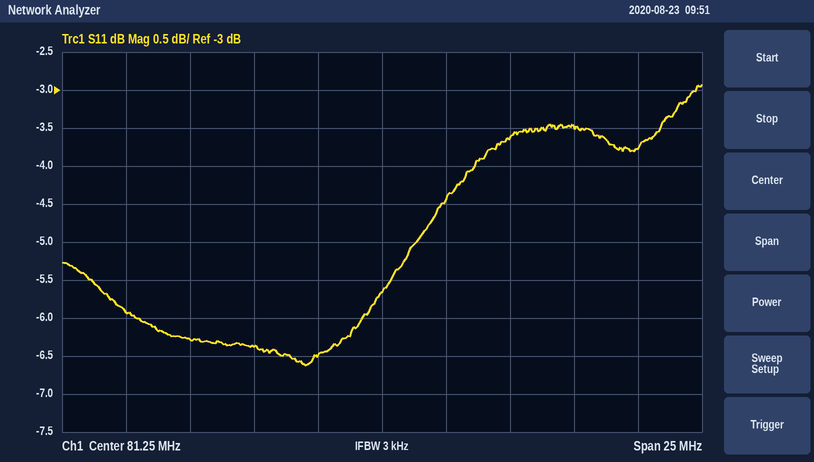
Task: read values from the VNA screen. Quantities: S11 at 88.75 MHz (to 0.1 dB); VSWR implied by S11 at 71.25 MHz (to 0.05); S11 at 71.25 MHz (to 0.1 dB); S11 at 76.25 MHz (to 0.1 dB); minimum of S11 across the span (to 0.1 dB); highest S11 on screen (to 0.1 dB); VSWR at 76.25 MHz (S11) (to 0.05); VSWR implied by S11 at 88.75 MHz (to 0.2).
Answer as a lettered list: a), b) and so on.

a) -3.5 dB
b) 3.05
c) -5.9 dB
d) -6.4 dB
e) -6.6 dB
f) -2.9 dB
g) 2.85
h) 5.0
